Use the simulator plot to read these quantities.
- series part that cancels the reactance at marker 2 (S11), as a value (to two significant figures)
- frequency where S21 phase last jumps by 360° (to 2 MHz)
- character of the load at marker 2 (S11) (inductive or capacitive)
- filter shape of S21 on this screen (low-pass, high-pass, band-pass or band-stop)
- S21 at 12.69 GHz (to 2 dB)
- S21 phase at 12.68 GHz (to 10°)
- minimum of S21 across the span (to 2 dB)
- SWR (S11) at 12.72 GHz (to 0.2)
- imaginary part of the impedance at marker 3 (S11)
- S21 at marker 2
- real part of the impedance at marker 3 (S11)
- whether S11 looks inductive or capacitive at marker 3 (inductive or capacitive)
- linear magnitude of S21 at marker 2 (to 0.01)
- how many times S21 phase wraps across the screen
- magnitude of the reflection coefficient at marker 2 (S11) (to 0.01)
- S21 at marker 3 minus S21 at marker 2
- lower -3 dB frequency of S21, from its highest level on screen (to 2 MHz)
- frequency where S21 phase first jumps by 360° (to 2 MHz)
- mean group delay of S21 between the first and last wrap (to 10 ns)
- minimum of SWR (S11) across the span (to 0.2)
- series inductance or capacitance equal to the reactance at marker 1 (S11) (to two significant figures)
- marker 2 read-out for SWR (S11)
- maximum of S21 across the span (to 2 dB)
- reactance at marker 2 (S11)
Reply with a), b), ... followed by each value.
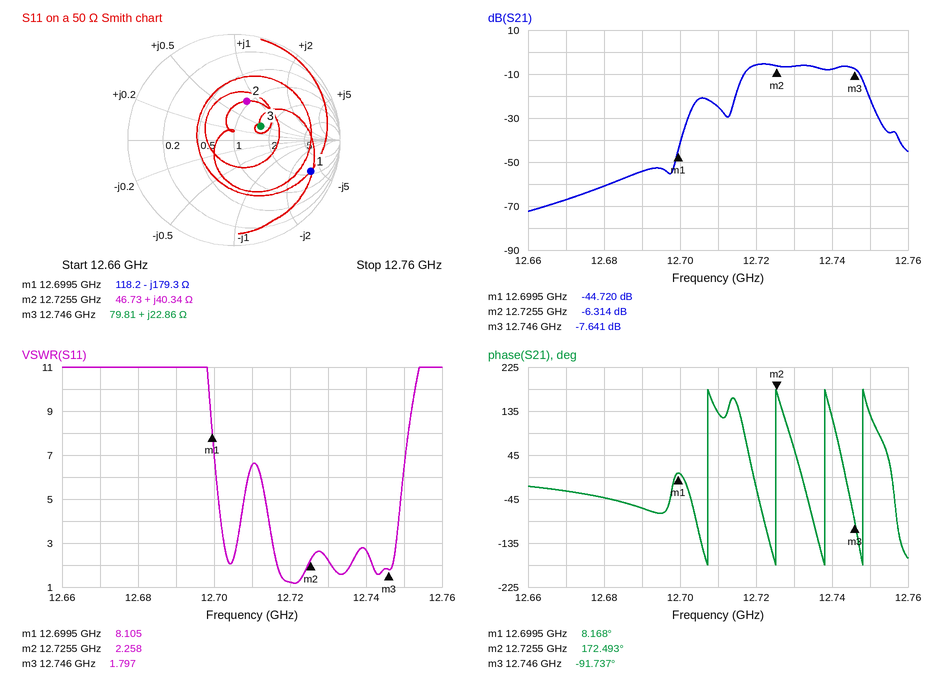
a) 310 fF
b) 12.748 GHz
c) inductive
d) band-pass
e) -54 dB
f) -40°
g) -72 dB
h) 1.2
i) +22.86 Ω
j) -6.314 dB
k) 79.81 Ω
l) inductive
m) 0.48
n) 4
o) 0.39
p) -1.327 dB
q) 12.718 GHz
r) 12.708 GHz
s) 70 ns
t) 1.2
u) 70 fF
v) 2.258
w) -6 dB
x) +40.34 Ω
